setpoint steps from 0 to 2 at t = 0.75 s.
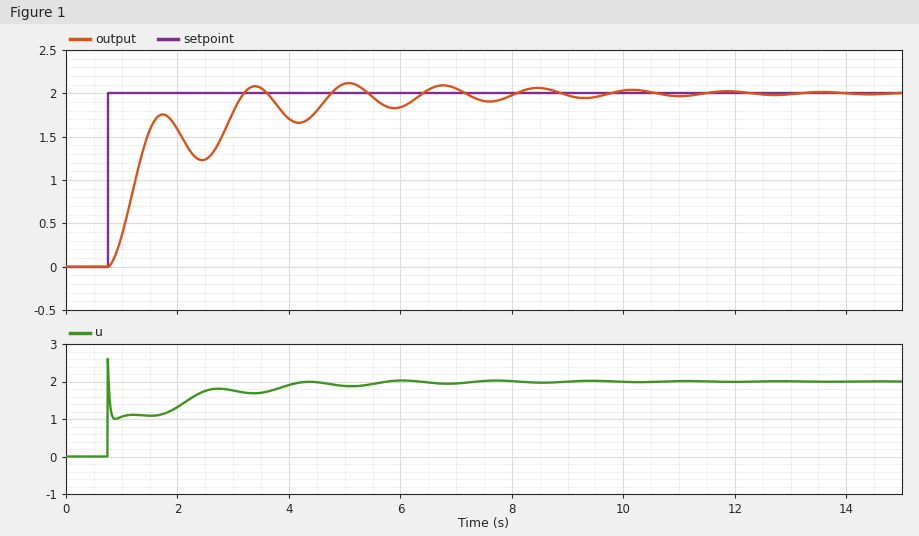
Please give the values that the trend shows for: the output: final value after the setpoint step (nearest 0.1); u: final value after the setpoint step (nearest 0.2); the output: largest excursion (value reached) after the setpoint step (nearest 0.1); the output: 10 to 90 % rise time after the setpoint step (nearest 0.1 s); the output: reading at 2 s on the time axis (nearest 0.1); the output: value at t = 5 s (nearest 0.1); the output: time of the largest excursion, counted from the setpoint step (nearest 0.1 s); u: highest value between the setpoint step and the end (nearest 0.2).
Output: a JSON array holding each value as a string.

["2.0", "2.0", "2.1", "2.1 s", "1.6", "2.1", "4.3 s", "2.6"]
